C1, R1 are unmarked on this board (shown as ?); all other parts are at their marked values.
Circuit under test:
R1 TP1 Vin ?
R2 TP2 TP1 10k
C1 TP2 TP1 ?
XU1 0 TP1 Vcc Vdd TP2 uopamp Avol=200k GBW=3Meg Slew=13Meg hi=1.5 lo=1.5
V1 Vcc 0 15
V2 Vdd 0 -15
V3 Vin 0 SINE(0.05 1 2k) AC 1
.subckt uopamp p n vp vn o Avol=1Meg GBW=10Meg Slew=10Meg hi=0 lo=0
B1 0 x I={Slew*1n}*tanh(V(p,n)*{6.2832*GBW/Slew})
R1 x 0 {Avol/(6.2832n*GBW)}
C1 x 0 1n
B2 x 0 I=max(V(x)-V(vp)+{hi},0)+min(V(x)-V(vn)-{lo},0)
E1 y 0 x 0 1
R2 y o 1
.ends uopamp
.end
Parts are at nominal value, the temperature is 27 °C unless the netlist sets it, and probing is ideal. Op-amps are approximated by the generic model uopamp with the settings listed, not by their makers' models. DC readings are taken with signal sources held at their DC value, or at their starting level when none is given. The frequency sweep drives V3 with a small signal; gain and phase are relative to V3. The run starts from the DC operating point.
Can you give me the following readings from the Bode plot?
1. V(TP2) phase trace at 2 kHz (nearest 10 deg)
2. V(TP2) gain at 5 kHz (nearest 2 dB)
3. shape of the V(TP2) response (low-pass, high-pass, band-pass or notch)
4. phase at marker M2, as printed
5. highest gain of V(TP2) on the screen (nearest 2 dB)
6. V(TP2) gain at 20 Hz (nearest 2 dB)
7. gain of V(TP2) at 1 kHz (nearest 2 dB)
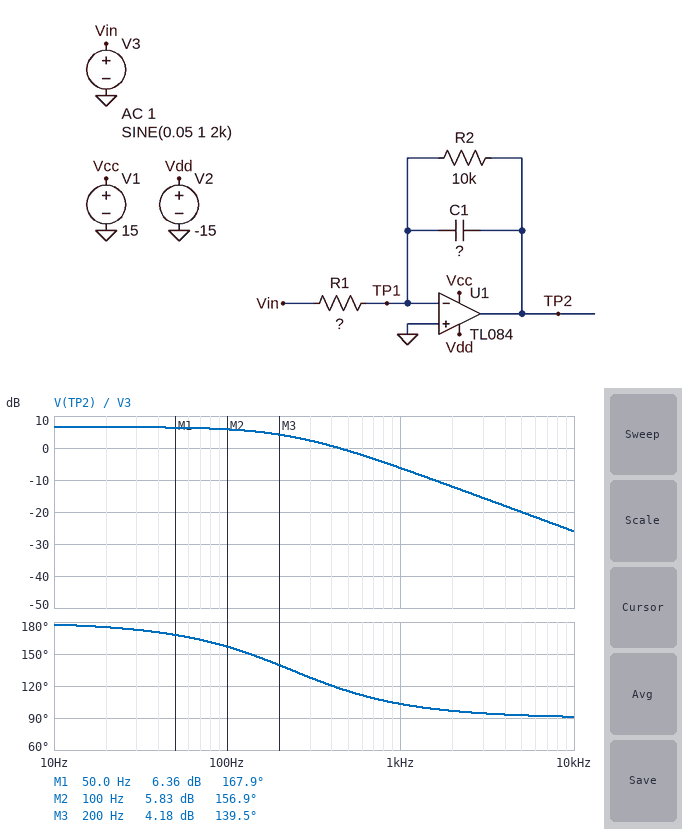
100 deg
-20 dB
low-pass
156.9 deg
6 dB
6 dB
-6 dB
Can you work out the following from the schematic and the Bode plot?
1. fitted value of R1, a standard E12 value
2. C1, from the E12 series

4.7 kΩ
68 nF
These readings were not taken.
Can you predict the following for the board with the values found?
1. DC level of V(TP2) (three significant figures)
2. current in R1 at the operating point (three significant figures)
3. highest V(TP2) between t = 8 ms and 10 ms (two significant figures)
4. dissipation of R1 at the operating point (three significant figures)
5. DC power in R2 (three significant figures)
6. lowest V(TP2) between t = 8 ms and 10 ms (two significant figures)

-106 mV
10.6 µA
140 mV
532 nW
1.13 µW
-350 mV
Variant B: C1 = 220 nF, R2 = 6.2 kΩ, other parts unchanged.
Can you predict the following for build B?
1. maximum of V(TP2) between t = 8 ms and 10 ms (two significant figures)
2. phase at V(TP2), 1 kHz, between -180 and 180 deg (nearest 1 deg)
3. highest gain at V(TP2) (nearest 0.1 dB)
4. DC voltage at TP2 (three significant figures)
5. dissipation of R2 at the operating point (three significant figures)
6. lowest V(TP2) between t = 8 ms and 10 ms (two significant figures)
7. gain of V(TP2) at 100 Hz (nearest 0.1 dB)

11 mV
97 deg
2.4 dB
-66.0 mV
702 nW
-140 mV
0 dB
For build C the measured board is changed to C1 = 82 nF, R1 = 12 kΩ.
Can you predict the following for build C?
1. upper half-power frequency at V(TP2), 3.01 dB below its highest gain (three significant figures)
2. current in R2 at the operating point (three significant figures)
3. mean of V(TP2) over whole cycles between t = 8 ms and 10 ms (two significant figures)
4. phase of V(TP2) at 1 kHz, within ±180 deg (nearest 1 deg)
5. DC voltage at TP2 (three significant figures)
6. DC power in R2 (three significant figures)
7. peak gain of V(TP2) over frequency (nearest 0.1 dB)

194 Hz
4.17 µA
-42 mV
101 deg
-41.7 mV
174 nW
-1.6 dB
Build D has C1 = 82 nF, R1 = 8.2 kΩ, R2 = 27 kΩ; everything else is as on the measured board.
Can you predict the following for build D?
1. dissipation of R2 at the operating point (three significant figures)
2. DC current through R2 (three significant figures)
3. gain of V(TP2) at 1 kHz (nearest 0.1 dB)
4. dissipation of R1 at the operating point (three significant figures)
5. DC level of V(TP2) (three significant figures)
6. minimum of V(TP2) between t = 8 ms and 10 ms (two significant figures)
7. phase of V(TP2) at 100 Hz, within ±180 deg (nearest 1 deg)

1.00 µW
6.10 µA
-12.5 dB
305 nW
-165 mV
-290 mV
126 deg
